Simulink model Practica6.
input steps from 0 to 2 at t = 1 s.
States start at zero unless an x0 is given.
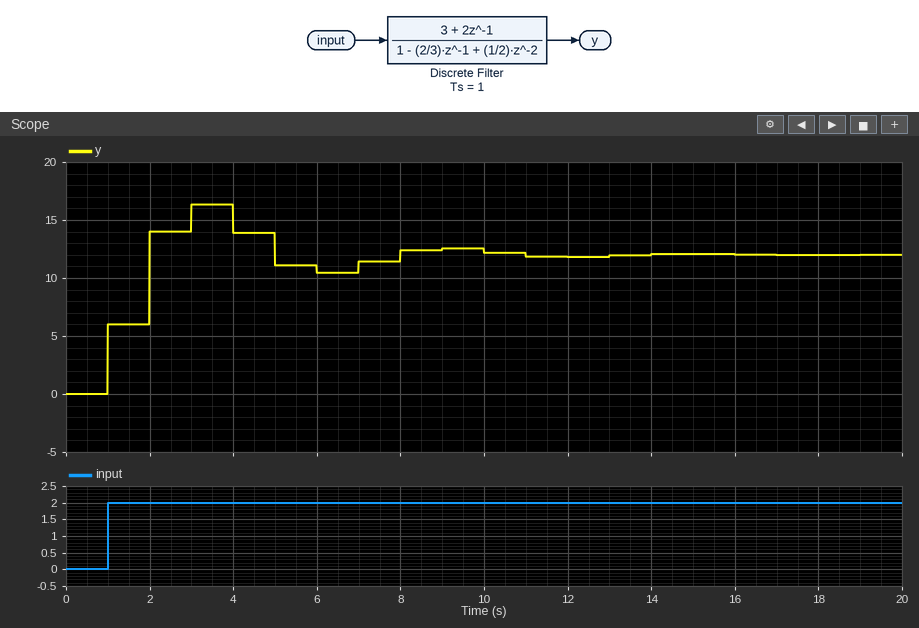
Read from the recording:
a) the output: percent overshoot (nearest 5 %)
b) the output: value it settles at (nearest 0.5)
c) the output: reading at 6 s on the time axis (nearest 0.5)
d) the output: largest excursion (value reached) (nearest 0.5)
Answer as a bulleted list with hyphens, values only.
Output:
- 35 %
- 12.0
- 10.5
- 16.5
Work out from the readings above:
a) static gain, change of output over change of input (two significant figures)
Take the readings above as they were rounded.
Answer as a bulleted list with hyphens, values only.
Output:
- 6.0
